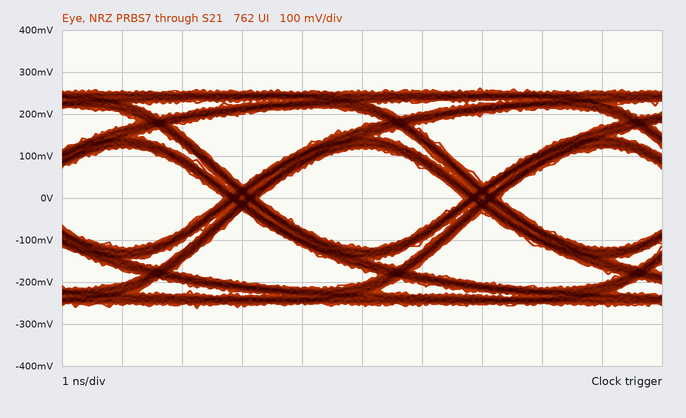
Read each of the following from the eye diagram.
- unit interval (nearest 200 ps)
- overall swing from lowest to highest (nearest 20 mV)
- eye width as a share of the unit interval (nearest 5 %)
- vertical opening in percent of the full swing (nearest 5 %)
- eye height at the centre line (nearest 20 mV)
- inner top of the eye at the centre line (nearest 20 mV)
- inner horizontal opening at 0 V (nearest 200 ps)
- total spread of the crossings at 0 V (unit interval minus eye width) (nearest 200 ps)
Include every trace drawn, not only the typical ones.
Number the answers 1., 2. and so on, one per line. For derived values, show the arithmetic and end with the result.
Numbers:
1. 4.0 ns
2. 520 mV
3. 3.4 ns / 4.0 ns ≈ 85 %
4. 240 mV / 520 mV ≈ 46.2 %, so 45 % to the nearest 5 %
5. 240 mV
6. 120 mV
7. 3.4 ns
8. 600 ps
